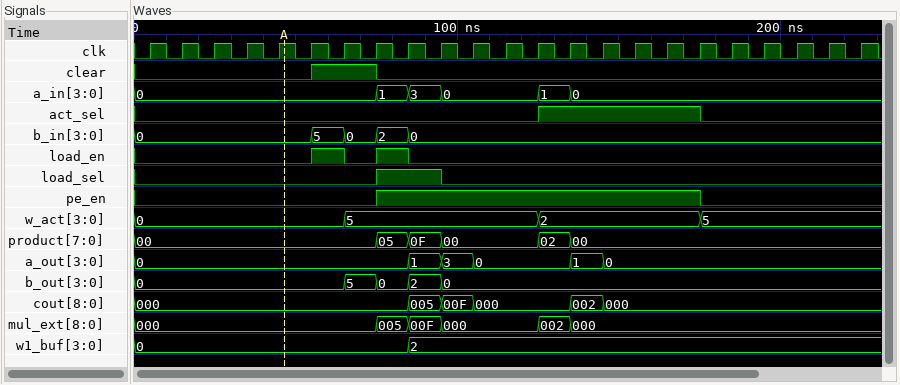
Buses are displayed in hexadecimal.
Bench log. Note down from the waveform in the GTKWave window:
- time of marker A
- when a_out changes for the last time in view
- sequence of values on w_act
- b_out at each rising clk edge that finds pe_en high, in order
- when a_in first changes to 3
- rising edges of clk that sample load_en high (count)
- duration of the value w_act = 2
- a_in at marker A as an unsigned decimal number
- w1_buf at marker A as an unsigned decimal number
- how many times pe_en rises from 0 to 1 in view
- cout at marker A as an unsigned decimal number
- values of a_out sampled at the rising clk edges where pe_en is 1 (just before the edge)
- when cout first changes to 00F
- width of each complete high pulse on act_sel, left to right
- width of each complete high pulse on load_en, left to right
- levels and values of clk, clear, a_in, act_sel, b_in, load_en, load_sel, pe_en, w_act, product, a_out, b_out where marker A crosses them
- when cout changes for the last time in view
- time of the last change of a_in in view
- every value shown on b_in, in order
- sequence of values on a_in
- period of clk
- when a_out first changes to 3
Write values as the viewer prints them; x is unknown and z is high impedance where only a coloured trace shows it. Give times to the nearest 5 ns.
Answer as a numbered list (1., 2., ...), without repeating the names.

1. 45 ns
2. 145 ns
3. 0, 5, 2, 5
4. 0, 2, 0, 0, 0, 0, 0, 0, 0, 0
5. 85 ns
6. 2
7. 50 ns
8. 0
9. 0
10. 1
11. 0
12. 0, 1, 3, 0, 0, 0, 1, 0, 0, 0
13. 95 ns
14. 50 ns
15. 10 ns, 10 ns
16. clk=1, clear=0, a_in=0, act_sel=0, b_in=0, load_en=0, load_sel=0, pe_en=0, w_act=0, product=00, a_out=0, b_out=0
17. 145 ns
18. 135 ns
19. 0, 5, 0, 2, 0
20. 0, 1, 3, 0, 1, 0
21. 10 ns
22. 95 ns
